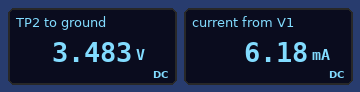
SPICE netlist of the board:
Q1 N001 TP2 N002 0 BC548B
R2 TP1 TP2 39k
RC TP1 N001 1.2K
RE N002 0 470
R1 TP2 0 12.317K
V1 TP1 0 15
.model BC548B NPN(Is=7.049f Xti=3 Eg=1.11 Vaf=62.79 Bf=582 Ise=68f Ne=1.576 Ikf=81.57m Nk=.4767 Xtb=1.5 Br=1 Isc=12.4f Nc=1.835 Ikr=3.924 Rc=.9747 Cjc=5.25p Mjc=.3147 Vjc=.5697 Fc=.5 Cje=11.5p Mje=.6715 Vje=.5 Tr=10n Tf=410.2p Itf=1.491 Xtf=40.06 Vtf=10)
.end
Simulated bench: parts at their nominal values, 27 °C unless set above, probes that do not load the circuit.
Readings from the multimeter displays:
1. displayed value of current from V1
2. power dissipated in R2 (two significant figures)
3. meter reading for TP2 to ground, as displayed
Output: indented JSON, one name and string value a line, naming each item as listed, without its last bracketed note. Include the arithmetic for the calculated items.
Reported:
{
  "displayed value of current from V1": "6.18 mA",
  "power dissipated in R2": "(15 V - 3.483 V)^2 / 39 kΩ = 3.4 mW",
  "meter reading for TP2 to ground, as displayed": "3.483 V"
}
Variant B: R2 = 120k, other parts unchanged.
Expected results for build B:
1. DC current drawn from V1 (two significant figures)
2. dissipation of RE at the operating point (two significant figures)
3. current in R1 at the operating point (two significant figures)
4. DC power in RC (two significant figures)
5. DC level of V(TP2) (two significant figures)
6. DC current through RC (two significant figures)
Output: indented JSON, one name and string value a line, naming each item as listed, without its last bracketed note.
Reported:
{
  "DC current drawn from V1": "1.6 mA",
  "dissipation of RE at the operating point": "1.0 mW",
  "current in R1 at the operating point": "110 µA",
  "DC power in RC": "2.6 mW",
  "DC level of V(TP2)": "1.4 V",
  "DC current through RC": "1.5 mA"
}
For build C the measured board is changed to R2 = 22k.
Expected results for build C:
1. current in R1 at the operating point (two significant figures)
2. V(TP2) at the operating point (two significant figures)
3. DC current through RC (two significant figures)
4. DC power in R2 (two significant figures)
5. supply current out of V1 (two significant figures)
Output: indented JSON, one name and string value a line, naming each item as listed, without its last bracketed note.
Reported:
{
  "current in R1 at the operating point": "400 µA",
  "V(TP2) at the operating point": "4.9 V",
  "DC current through RC": "8.9 mA",
  "DC power in R2": "4.6 mW",
  "supply current out of V1": "9.3 mA"
}
